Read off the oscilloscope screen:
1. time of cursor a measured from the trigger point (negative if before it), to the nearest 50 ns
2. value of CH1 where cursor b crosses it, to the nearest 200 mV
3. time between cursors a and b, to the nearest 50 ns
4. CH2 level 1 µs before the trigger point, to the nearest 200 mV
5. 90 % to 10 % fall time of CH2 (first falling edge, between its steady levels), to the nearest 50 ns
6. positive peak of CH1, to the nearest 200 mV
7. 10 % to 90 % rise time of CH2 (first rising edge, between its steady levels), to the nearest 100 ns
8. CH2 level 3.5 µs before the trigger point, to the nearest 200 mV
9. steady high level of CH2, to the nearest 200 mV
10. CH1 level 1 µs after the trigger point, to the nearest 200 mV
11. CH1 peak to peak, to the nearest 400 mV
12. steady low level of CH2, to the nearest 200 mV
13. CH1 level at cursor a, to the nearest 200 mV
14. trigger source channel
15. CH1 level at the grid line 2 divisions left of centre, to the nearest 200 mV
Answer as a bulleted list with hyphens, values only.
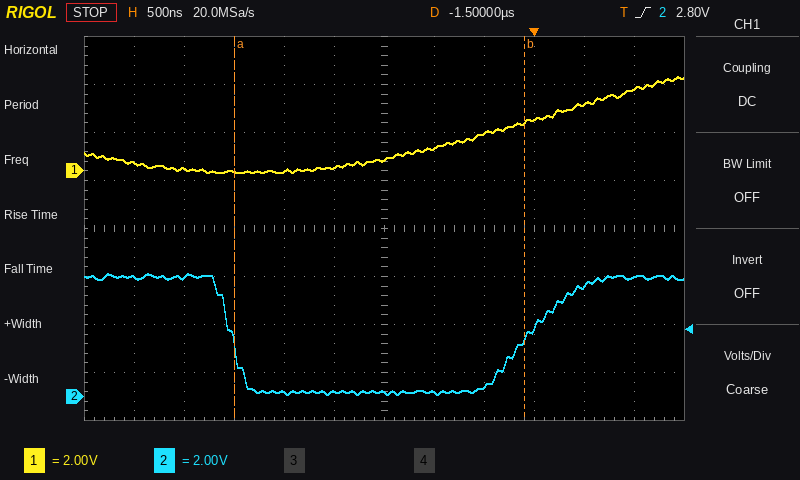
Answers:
- -3.00 µs
- 2.0 V
- 2.90 µs
- 200 mV
- 300 ns
- 4.0 V
- 800 ns
- 5.0 V
- 5.0 V
- 3.4 V
- 4.0 V
- 200 mV
- 0.0 V
- CH2
- 0.0 V
